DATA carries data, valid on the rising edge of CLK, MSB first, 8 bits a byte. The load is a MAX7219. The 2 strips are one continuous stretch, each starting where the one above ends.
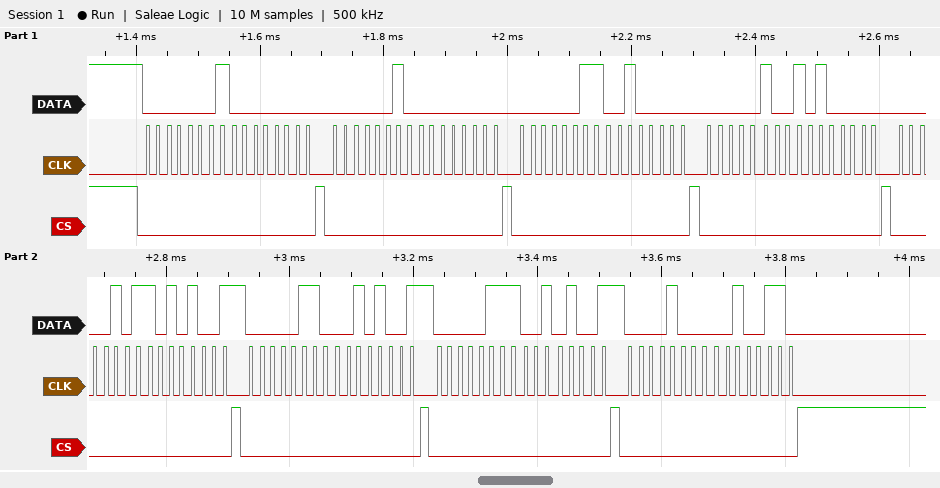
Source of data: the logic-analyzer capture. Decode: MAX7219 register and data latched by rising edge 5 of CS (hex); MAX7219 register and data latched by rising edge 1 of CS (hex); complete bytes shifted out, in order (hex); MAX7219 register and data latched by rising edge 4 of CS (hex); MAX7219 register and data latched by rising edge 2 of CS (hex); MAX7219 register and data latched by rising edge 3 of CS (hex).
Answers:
register 0x5, data 0xA9
register 0x1, data 0x00
01 00 02 00 03 20 04 A0 05 A9 06 29 07 29 08 26
register 0x4, data 0xA0
register 0x2, data 0x00
register 0x3, data 0x20
